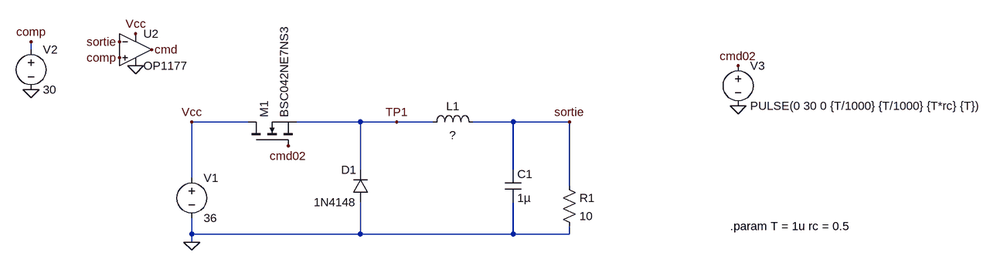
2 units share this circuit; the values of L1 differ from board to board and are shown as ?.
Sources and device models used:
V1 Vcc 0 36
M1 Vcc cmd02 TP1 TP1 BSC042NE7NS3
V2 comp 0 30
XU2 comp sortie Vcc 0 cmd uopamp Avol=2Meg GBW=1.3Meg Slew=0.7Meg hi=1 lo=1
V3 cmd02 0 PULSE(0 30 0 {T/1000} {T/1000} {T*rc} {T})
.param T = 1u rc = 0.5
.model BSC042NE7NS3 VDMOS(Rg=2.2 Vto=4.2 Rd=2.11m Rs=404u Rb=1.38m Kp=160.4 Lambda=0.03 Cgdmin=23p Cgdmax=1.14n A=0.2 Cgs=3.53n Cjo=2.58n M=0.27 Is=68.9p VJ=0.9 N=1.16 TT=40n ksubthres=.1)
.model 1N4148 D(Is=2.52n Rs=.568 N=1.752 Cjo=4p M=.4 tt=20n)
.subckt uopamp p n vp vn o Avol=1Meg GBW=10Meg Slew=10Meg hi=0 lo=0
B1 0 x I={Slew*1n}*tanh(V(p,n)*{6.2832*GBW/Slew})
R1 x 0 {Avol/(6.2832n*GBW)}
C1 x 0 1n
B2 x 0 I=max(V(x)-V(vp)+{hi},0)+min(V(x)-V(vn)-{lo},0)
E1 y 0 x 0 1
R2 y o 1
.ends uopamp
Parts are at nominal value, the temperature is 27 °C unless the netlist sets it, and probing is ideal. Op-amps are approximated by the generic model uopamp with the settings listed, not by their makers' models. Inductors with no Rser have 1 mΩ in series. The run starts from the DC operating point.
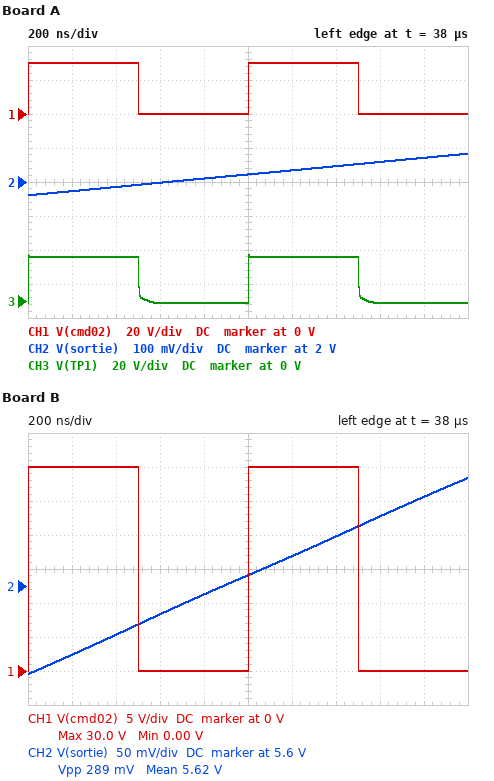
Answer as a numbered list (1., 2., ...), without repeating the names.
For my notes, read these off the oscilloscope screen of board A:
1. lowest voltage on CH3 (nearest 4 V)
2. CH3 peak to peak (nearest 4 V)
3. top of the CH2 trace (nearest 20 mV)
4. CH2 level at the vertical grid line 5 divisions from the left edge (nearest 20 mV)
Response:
1. 0 V
2. 28 V
3. 2.08 V
4. 2.02 V
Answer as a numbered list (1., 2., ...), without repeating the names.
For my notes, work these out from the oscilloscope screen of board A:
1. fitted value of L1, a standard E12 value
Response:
1. 1.8 mH
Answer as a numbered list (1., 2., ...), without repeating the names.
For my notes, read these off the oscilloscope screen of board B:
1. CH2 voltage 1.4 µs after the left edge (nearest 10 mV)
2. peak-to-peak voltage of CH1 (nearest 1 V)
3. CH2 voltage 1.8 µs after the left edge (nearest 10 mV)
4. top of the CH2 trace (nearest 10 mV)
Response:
1. 5.67 V
2. 30 V
3. 5.73 V
4. 5.76 V
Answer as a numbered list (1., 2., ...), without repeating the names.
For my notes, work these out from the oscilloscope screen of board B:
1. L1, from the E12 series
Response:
1. 560 µH
